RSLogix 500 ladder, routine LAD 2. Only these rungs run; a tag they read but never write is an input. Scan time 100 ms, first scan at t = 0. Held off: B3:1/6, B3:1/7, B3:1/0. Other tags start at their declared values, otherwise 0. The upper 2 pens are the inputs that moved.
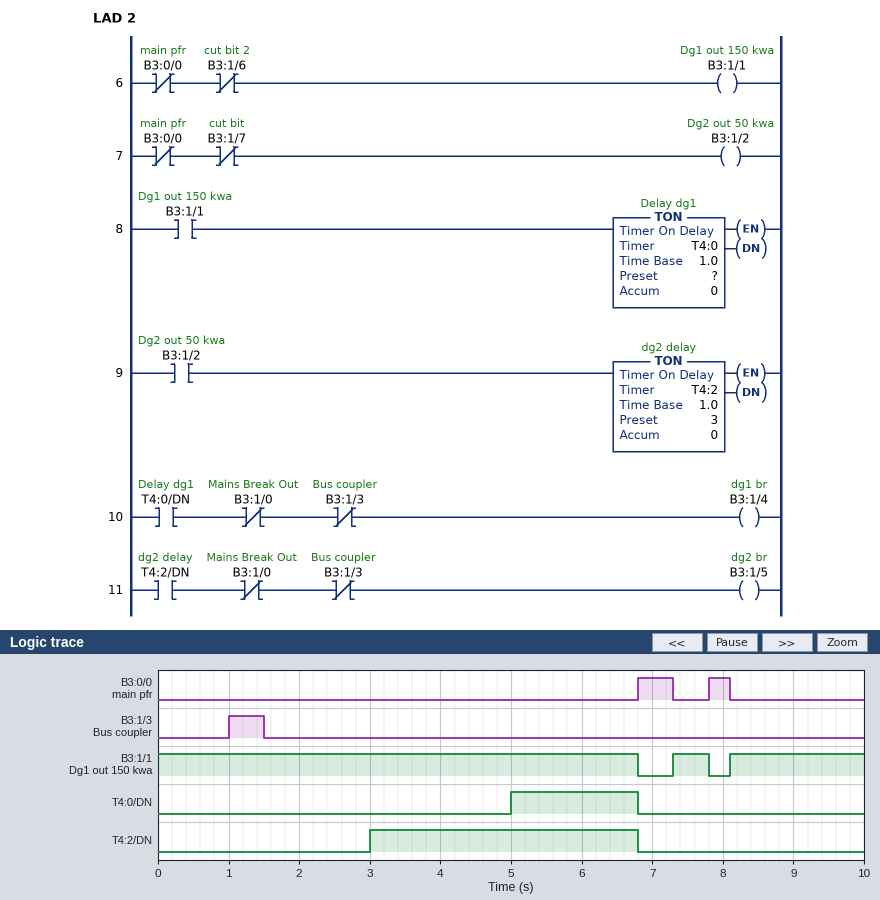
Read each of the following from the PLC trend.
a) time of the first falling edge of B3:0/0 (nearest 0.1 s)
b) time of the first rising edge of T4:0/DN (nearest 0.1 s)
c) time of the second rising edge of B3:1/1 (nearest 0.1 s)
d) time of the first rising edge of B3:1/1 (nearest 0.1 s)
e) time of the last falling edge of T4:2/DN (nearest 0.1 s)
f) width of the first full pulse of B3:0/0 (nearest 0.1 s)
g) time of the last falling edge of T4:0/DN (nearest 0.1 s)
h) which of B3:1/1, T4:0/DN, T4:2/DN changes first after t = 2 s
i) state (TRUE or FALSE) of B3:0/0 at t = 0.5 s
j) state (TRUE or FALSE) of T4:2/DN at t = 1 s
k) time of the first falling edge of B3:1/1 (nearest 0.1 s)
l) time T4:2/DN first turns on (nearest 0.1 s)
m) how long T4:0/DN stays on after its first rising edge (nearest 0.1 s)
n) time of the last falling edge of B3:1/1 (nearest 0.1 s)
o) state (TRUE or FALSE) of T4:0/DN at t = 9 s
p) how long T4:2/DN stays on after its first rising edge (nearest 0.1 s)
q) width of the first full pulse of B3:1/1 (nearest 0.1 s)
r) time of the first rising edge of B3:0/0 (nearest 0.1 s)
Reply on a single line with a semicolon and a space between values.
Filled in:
7.3 s; 5.0 s; 8.1 s; 7.3 s; 6.8 s; 0.5 s; 6.8 s; T4:2/DN; FALSE; FALSE; 6.8 s; 3.0 s; 1.8 s; 7.8 s; FALSE; 3.8 s; 0.5 s; 6.8 s
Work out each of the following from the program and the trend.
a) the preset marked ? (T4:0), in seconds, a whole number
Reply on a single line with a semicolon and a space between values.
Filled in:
5 s
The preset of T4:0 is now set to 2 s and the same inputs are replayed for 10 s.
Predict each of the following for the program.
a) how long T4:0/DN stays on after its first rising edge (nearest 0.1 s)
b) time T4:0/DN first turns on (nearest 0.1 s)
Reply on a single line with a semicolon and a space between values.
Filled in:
4.8 s; 2.0 s
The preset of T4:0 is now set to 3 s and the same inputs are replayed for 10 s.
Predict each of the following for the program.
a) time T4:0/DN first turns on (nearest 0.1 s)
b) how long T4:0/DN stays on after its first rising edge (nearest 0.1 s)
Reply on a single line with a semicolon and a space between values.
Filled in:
3.0 s; 3.8 s
